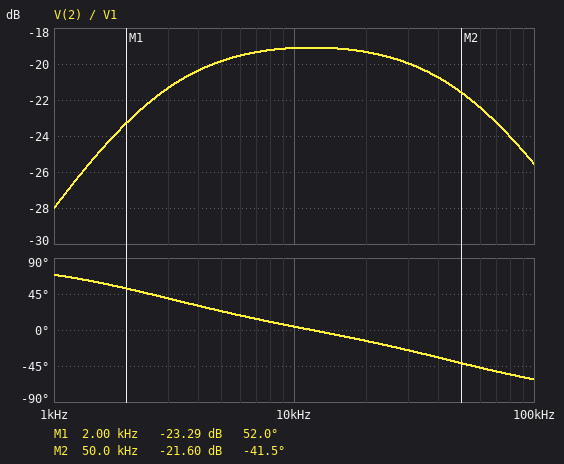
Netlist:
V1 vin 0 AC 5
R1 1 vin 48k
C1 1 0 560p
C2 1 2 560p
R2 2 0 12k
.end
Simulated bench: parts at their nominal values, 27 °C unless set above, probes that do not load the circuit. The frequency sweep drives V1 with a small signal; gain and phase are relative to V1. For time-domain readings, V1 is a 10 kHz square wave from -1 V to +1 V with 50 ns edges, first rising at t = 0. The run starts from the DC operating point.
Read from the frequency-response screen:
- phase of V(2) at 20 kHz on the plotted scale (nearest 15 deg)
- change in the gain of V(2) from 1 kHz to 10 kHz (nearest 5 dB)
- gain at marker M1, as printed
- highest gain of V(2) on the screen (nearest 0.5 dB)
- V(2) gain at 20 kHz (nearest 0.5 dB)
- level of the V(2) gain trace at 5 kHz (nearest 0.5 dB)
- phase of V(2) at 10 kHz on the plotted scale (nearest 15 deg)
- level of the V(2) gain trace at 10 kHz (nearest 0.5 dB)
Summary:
-15 deg
10 dB
-23.29 dB
-19.0 dB
-19.5 dB
-20.0 dB
0 deg
-19.0 dB
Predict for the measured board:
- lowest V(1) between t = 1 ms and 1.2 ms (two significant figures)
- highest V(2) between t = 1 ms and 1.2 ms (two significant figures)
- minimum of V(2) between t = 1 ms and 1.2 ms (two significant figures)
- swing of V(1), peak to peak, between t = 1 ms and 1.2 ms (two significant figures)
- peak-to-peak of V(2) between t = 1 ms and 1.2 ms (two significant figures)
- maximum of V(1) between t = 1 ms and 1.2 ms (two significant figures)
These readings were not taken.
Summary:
-450 mV
140 mV
-140 mV
900 mV
270 mV
450 mV
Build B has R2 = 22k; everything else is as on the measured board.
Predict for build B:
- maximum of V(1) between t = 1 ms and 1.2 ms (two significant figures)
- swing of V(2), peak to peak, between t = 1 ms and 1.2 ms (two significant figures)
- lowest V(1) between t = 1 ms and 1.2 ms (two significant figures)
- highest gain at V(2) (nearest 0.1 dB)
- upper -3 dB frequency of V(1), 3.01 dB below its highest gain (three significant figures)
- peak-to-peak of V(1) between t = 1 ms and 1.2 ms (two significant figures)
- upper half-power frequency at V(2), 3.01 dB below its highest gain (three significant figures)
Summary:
470 mV
430 mV
-470 mV
-14.6 dB
2.72 kHz
930 mV
34.0 kHz
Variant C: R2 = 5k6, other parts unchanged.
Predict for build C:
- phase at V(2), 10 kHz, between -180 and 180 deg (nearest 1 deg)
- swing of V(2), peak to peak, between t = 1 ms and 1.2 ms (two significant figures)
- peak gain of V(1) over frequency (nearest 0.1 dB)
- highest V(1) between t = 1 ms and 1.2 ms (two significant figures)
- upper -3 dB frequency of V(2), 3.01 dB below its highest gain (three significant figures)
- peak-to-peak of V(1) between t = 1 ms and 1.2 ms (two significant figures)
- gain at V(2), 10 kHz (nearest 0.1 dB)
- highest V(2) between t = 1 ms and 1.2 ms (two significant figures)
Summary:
11 deg
140 mV
0 dB
440 mV
110 kHz
880 mV
-25.3 dB
72 mV
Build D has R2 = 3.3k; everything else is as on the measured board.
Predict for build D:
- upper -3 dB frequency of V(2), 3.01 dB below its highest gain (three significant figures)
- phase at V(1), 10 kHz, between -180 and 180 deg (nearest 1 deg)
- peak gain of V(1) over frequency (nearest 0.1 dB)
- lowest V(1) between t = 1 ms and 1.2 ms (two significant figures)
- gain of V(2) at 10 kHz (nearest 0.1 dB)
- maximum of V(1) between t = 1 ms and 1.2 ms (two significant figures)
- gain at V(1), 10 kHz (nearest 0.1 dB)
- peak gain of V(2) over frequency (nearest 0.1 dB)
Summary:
181 kHz
-70 deg
0 dB
-440 mV
-29.8 dB
440 mV
-11.0 dB
-29.6 dB
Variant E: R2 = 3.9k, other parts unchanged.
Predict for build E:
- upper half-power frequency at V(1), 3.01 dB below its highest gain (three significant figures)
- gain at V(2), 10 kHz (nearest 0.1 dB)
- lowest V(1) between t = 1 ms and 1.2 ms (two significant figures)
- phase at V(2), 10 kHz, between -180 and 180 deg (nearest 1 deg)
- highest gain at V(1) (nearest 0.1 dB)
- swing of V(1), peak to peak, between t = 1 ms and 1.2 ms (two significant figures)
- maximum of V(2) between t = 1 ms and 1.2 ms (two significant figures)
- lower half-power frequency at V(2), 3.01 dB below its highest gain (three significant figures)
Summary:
2.90 kHz
-28.4 dB
-440 mV
12 deg
0 dB
880 mV
52 mV
2.79 kHz
